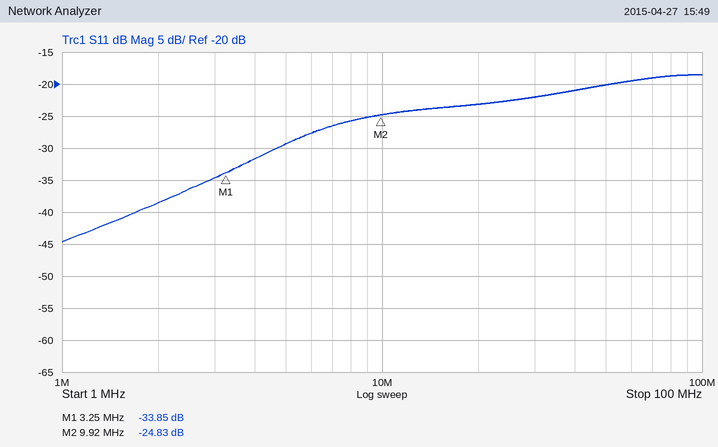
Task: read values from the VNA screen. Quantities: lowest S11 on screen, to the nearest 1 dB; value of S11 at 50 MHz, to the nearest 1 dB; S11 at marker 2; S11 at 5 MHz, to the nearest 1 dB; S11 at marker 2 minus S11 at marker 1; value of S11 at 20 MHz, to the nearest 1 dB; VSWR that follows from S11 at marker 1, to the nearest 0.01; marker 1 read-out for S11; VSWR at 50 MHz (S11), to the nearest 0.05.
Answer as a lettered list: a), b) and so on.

a) -45 dB
b) -20 dB
c) -24.83 dB
d) -29 dB
e) 9.02 dB
f) -23 dB
g) 1.04
h) -33.85 dB
i) 1.20
